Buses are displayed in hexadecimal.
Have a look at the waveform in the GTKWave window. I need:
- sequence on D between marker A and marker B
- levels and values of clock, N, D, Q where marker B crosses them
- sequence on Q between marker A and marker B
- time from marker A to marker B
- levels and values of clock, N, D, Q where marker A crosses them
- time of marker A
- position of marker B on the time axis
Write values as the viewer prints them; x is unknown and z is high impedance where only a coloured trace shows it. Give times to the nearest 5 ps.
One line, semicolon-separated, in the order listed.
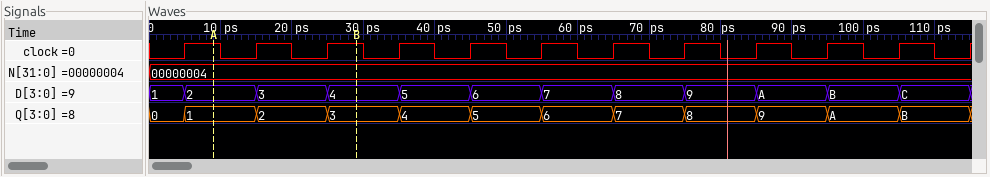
2, 3, 4; clock=1, N=00000004, D=4, Q=3; 1, 2, 3; 20 ps; clock=1, N=00000004, D=2, Q=1; 10 ps; 30 ps
